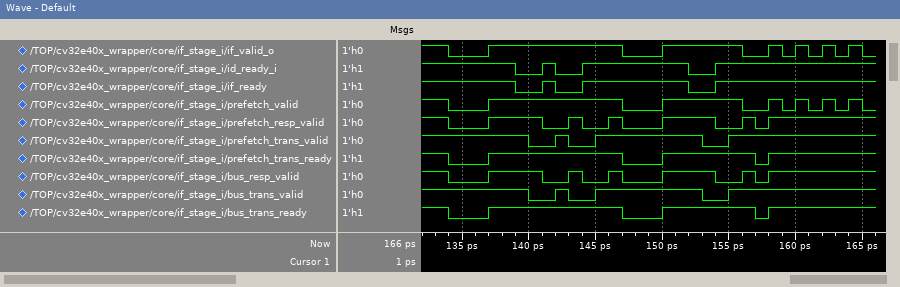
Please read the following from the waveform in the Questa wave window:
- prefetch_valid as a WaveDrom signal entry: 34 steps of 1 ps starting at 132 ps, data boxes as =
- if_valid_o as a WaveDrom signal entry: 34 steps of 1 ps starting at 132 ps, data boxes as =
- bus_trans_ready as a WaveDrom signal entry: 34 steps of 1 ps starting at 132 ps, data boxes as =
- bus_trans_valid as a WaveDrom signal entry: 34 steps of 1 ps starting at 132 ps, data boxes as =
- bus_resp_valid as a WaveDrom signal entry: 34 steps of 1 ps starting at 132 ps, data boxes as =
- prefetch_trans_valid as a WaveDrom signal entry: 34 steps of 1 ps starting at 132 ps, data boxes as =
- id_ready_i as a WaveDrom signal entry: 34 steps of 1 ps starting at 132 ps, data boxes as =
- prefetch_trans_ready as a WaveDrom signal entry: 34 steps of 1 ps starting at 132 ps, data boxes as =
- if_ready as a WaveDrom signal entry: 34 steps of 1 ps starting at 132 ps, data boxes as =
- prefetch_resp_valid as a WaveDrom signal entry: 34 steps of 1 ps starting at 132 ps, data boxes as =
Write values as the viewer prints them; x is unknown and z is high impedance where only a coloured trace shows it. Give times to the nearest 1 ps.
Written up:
{name: 'prefetch_valid', wave: '1.0..1.........0..1.....0.10101010'}
{name: 'if_valid_o', wave: '1.0..1.........0..1.....0.10101010'}
{name: 'bus_trans_ready', wave: '1.0..1.........0..1......01.......'}
{name: 'bus_trans_valid', wave: '1.......0.10.1.......0.1..........'}
{name: 'bus_resp_valid', wave: '1.0..1...0.10.10..1...0.101.......'}
{name: 'prefetch_trans_valid', wave: '1.......0.10.1.......0.1..........'}
{name: 'id_ready_i', wave: '1......0.10.1.......0.1...........'}
{name: 'prefetch_trans_ready', wave: '1.0..1.........0..1......01.......'}
{name: 'if_ready', wave: '1......0.10.1.......0.1...........'}
{name: 'prefetch_resp_valid', wave: '1.0..1...0.10.10..1...0.101.......'}
